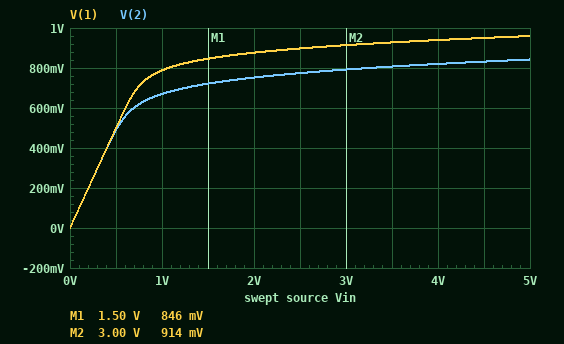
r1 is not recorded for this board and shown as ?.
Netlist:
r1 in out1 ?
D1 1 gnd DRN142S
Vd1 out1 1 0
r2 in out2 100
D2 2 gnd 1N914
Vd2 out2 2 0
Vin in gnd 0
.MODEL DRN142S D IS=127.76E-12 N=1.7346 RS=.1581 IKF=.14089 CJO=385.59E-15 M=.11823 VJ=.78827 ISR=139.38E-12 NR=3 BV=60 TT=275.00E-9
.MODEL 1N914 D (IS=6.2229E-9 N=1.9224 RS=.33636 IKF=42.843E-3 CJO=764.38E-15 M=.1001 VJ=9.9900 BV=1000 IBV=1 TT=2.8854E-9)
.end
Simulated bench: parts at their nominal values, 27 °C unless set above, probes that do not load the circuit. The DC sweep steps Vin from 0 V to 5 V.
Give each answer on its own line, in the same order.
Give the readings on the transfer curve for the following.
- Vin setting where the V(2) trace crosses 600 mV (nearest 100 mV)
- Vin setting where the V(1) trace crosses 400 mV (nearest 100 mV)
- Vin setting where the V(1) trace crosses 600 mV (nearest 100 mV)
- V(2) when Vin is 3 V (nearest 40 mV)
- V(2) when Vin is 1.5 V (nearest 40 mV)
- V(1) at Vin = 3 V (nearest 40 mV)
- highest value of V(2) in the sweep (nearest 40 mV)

700 mV
400 mV
600 mV
800 mV
720 mV
920 mV
840 mV
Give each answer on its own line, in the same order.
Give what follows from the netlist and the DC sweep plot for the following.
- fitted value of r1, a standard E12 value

47 Ω
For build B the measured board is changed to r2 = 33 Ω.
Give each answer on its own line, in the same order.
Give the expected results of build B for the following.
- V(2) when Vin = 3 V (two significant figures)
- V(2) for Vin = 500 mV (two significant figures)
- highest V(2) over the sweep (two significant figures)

880 mV
500 mV
950 mV
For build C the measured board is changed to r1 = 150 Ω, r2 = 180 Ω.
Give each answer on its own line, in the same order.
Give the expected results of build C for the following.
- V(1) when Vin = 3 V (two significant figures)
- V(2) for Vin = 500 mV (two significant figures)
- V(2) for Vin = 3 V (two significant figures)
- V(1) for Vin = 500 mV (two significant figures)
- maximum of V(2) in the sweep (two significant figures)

850 mV
480 mV
750 mV
500 mV
800 mV
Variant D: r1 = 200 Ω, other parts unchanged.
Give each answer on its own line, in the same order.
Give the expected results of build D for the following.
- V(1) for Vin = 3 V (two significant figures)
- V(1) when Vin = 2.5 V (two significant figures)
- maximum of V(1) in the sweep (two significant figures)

830 mV
820 mV
870 mV
